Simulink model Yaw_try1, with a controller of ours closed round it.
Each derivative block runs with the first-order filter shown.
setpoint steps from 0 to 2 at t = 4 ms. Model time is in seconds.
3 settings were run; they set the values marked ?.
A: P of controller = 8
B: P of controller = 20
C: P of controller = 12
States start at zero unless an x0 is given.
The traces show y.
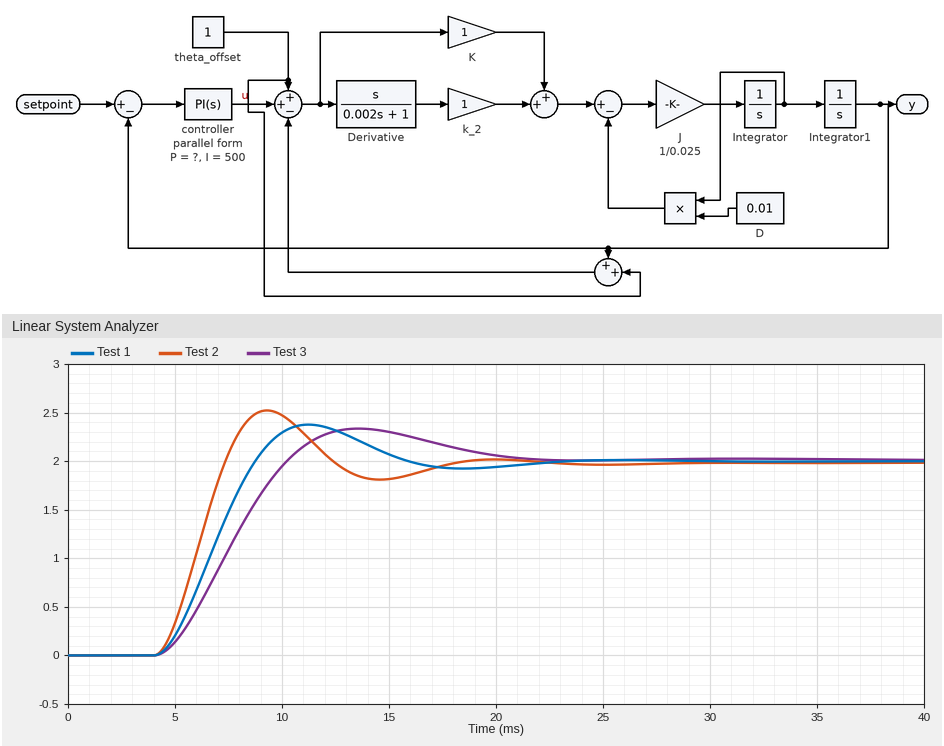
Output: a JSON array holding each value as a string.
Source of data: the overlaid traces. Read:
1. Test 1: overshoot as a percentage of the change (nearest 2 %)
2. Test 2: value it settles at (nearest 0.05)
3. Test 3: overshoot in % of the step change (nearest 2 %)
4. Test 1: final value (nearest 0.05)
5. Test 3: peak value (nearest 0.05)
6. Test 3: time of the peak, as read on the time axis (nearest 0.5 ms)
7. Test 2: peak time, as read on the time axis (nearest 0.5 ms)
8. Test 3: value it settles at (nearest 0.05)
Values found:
["18 %", "2.00", "16 %", "2.00", "2.35", "13.5 ms", "9.5 ms", "2.00"]
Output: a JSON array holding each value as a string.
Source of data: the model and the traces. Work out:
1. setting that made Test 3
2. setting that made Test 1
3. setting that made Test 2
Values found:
["A", "C", "B"]
